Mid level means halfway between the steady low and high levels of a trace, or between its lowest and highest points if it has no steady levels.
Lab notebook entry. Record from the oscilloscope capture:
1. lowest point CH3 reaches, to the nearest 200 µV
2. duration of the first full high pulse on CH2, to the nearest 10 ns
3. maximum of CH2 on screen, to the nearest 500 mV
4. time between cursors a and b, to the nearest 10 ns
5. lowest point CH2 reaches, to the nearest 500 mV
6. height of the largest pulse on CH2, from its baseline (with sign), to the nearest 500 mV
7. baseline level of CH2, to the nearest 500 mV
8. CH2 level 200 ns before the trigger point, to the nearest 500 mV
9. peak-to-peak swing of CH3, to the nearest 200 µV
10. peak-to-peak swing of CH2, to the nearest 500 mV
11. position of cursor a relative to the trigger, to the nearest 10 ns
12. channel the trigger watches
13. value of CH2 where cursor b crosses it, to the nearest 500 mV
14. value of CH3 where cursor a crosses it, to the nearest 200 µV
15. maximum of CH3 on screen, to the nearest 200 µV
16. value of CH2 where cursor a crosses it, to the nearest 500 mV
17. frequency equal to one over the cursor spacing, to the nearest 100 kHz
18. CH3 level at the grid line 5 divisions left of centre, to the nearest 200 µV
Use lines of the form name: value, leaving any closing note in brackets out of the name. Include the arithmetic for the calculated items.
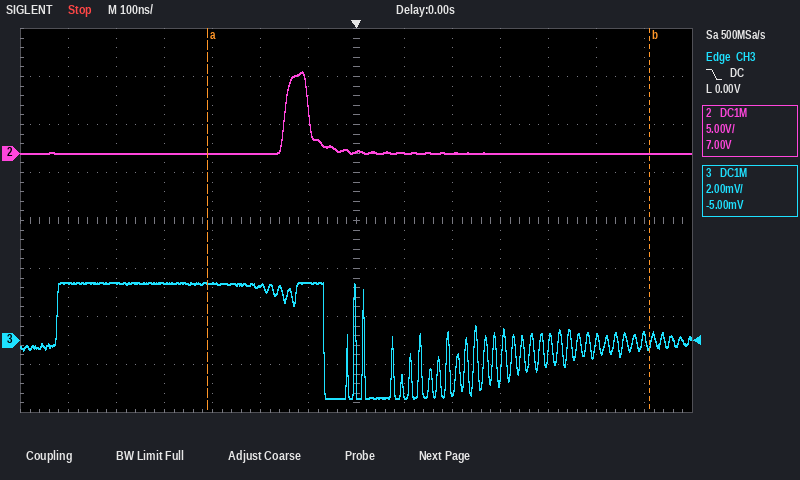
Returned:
lowest point CH3 reaches, to the nearest 200 µV: -2.4 mV
duration of the first full high pulse on CH2, to the nearest 10 ns: 50 ns
maximum of CH2 on screen, to the nearest 500 mV: 8.5 V
time between cursors a and b, to the nearest 10 ns: 920 ns
lowest point CH2 reaches, to the nearest 500 mV: 0.0 V
height of the largest pulse on CH2, from its baseline (with sign), to the nearest 500 mV: 8.5 V − (0.0 V) = +8.5 V
baseline level of CH2, to the nearest 500 mV: 0.0 V
CH2 level 200 ns before the trigger point, to the nearest 500 mV: 0.0 V
peak-to-peak swing of CH3, to the nearest 200 µV: 2.4 mV − (-2.4 mV) = 4.8 mV
peak-to-peak swing of CH2, to the nearest 500 mV: 8.5 V − (0.0 V) = 8.5 V
position of cursor a relative to the trigger, to the nearest 10 ns: -310 ns
channel the trigger watches: CH3
value of CH2 where cursor b crosses it, to the nearest 500 mV: 0.0 V
value of CH3 where cursor a crosses it, to the nearest 200 µV: 2.4 mV
maximum of CH3 on screen, to the nearest 200 µV: 2.4 mV
value of CH2 where cursor a crosses it, to the nearest 500 mV: 0.0 V
frequency equal to one over the cursor spacing, to the nearest 100 kHz: 1 / 920 ns ≈ 1.1 MHz
CH3 level at the grid line 5 divisions left of centre, to the nearest 200 µV: 2.4 mV
